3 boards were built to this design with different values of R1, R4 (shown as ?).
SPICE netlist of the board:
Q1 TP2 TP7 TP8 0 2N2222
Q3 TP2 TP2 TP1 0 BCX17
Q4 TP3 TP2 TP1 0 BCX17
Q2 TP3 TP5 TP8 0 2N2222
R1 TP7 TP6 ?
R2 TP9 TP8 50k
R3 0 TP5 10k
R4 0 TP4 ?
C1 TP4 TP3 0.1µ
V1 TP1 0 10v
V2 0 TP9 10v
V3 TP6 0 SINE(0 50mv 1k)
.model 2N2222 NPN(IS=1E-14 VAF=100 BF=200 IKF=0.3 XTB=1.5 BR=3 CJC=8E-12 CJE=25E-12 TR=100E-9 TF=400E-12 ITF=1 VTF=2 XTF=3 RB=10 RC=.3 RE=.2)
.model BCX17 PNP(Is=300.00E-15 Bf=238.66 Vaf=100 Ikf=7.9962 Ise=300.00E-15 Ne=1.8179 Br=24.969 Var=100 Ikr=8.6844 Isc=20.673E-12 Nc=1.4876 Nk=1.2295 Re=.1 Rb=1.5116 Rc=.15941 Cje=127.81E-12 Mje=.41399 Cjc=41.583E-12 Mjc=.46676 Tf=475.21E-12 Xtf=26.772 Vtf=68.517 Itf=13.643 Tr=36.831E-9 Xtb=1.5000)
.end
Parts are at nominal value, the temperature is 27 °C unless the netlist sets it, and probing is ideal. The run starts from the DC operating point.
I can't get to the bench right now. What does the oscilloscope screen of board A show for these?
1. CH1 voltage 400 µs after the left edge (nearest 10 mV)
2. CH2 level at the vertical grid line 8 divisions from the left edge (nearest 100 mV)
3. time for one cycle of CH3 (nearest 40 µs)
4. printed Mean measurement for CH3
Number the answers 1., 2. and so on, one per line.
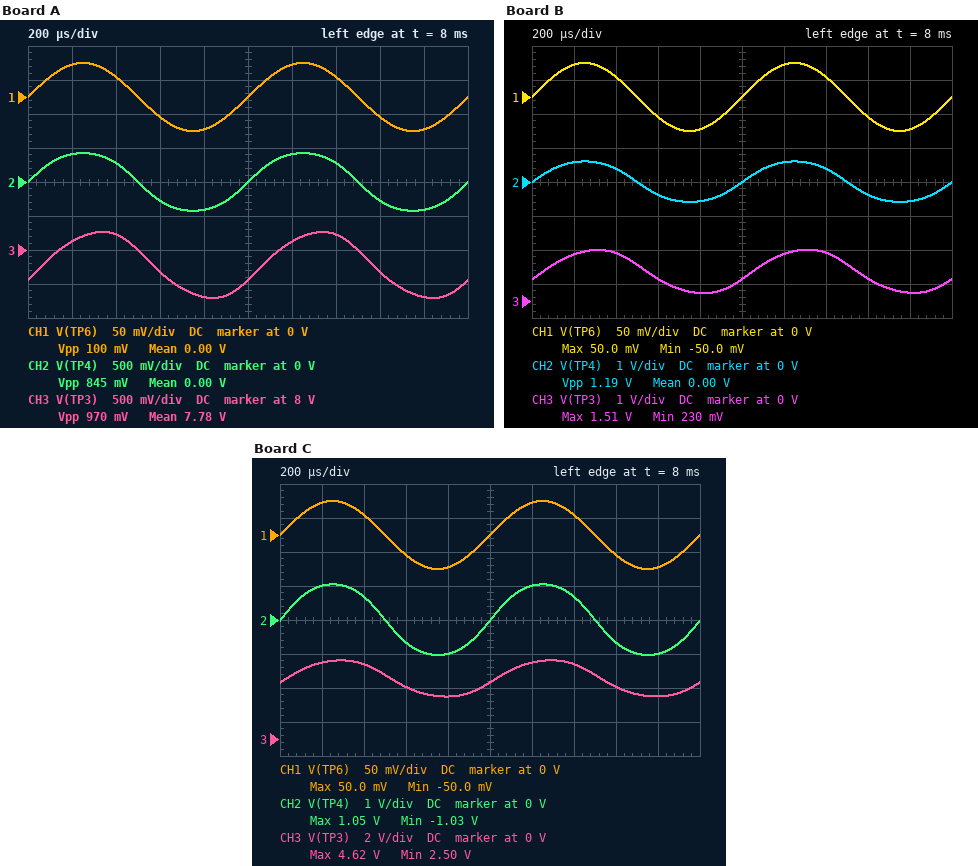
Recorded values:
1. 30 mV
2. -300 mV
3. 1.00 ms
4. 7.78 V
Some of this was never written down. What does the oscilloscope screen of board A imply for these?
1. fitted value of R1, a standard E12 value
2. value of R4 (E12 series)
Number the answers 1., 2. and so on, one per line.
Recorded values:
1. 12 kΩ
2. 3.3 kΩ
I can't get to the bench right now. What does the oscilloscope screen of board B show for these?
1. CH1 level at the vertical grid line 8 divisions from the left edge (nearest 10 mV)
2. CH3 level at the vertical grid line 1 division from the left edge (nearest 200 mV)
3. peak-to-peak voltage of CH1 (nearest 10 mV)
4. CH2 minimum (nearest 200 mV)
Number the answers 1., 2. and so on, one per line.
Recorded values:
1. -30 mV
2. 1.4 V
3. 100 mV
4. -600 mV
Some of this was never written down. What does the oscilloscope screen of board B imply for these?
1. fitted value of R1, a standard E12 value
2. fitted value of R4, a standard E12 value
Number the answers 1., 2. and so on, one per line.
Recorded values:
1. 22 kΩ
2. 4.7 kΩ
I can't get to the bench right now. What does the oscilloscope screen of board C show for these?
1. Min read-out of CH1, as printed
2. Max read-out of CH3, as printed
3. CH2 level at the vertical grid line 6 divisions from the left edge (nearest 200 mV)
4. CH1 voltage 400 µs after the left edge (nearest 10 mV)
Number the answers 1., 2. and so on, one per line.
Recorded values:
1. -50.0 mV
2. 4.62 V
3. 1.0 V
4. 30 mV
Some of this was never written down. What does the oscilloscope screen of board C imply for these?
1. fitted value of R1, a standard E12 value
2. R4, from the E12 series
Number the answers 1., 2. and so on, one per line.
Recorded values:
1. 18 kΩ
2. 8.2 kΩ
